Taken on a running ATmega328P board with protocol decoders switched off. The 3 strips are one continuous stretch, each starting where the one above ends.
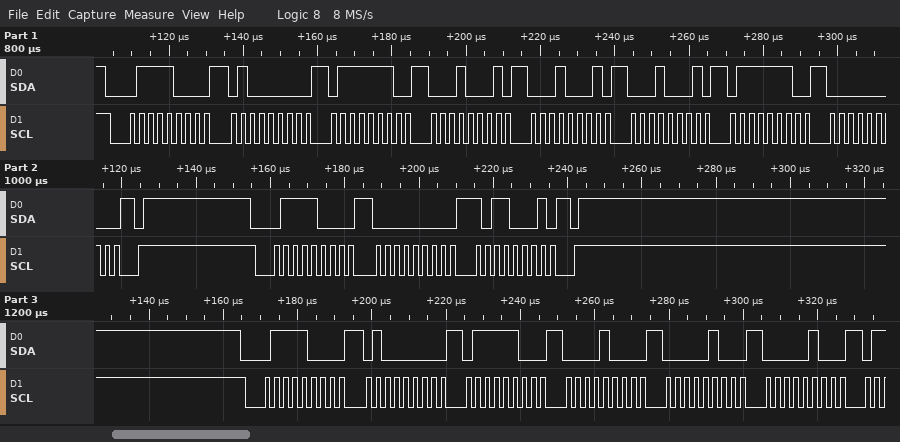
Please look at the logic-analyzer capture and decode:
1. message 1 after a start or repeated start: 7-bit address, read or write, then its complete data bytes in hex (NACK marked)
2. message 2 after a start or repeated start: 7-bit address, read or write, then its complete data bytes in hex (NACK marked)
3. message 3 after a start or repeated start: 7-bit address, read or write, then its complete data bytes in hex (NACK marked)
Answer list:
0x3C write: 40 7E 11 11 11 7E 00
0x3C write: 00 B1
0x3C write: 40 7C 08 04 04
